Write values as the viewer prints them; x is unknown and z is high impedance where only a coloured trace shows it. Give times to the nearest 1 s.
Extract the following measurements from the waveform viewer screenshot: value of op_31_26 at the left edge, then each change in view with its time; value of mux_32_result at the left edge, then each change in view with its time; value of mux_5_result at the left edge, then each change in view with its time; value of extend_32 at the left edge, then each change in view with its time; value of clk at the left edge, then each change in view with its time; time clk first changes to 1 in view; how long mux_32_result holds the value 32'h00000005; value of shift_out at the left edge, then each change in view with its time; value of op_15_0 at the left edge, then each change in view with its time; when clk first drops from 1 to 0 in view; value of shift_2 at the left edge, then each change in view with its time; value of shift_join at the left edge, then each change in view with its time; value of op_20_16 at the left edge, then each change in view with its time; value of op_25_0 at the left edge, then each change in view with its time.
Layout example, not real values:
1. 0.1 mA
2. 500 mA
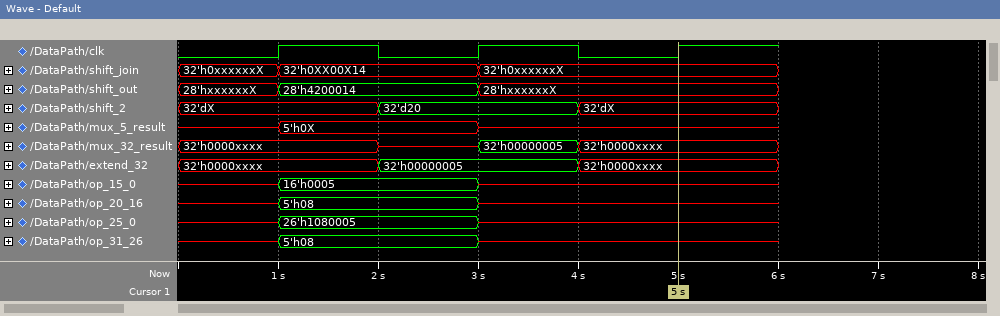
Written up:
1. x, 5'h08 at 1 s, x at 3 s
2. 32'h0000xxxx, x at 2 s, 32'h00000005 at 3 s, 32'h0000xxxx at 4 s
3. x, 5'h0X at 1 s, x at 3 s
4. 32'h0000xxxx, 32'h00000005 at 2 s, 32'h0000xxxx at 4 s
5. 0, 1 at 1 s, 0 at 2 s, 1 at 3 s, 0 at 4 s, 1 at 5 s
6. 1 s
7. 1 s
8. 28'hxxxxxxX, 28'h4200014 at 1 s, 28'hxxxxxxX at 3 s
9. x, 16'h0005 at 1 s, x at 3 s
10. 2 s
11. 32'dX, 32'd20 at 2 s, 32'dX at 4 s
12. 32'h0xxxxxxX, 32'h0XX00X14 at 1 s, 32'h0xxxxxxX at 3 s
13. x, 5'h08 at 1 s, x at 3 s
14. x, 26'h1080005 at 1 s, x at 3 s
